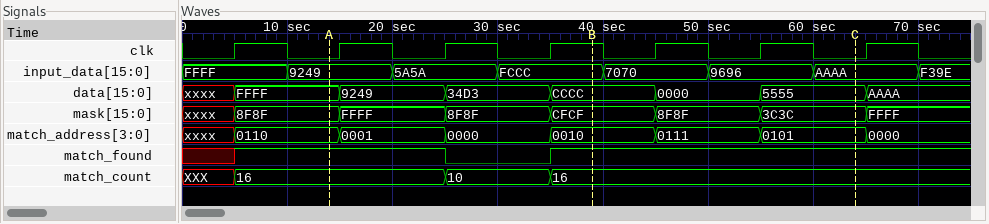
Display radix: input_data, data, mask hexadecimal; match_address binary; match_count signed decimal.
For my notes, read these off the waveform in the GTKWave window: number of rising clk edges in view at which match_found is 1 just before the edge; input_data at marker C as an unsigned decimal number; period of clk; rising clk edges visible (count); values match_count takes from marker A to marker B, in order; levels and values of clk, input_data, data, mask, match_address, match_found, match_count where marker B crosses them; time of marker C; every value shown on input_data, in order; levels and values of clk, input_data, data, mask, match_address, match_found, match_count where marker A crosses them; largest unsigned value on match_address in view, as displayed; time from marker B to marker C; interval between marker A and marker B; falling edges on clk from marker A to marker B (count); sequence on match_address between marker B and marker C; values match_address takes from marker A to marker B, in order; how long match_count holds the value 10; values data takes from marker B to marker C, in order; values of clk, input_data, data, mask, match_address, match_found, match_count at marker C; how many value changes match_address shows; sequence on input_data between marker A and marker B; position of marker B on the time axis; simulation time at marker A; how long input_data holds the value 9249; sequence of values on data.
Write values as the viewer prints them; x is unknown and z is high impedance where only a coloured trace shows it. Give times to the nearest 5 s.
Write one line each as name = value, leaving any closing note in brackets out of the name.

number of rising clk edges in view at which match_found is 1 just before the edge = 5
input_data at marker C as an unsigned decimal number = 43690
period of clk = 10 s
rising clk edges visible = 7
values match_count takes from marker A to marker B, in order = 16, 10, 16
levels and values of clk, input_data, data, mask, match_address, match_found, match_count where marker B crosses them = clk=1, input_data=FCCC, data=CCCC, mask=CFCF, match_address=0010, match_found=1, match_count=16
time of marker C = 65 s
every value shown on input_data, in order = FFFF, 9249, 5A5A, FCCC, 7070, 9696, AAAA, F39E
levels and values of clk, input_data, data, mask, match_address, match_found, match_count where marker A crosses them = clk=0, input_data=9249, data=FFFF, mask=8F8F, match_address=0110, match_found=1, match_count=16
largest unsigned value on match_address in view, as displayed = 0111
time from marker B to marker C = 25 s
interval between marker A and marker B = 25 s
falling edges on clk from marker A to marker B = 2
sequence on match_address between marker B and marker C = 0010, 0111, 0101
values match_address takes from marker A to marker B, in order = 0110, 0001, 0000, 0010
how long match_count holds the value 10 = 10 s
values data takes from marker B to marker C, in order = CCCC, 0000, 5555
values of clk, input_data, data, mask, match_address, match_found, match_count at marker C = clk=0, input_data=AAAA, data=5555, mask=3C3C, match_address=0101, match_found=1, match_count=16
how many value changes match_address shows = 7
sequence on input_data between marker A and marker B = 9249, 5A5A, FCCC
position of marker B on the time axis = 40 s
simulation time at marker A = 15 s
how long input_data holds the value 9249 = 10 s
sequence of values on data = xxxx, FFFF, 9249, 34D3, CCCC, 0000, 5555, AAAA
